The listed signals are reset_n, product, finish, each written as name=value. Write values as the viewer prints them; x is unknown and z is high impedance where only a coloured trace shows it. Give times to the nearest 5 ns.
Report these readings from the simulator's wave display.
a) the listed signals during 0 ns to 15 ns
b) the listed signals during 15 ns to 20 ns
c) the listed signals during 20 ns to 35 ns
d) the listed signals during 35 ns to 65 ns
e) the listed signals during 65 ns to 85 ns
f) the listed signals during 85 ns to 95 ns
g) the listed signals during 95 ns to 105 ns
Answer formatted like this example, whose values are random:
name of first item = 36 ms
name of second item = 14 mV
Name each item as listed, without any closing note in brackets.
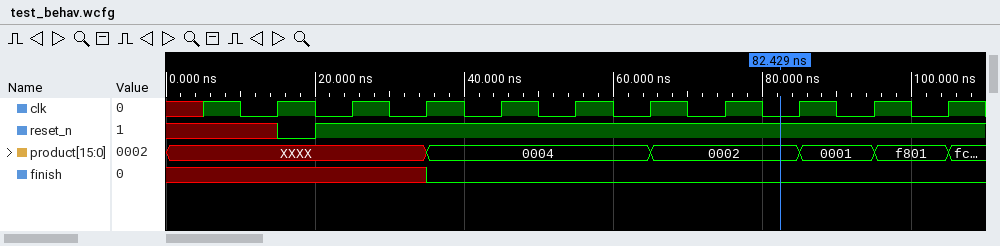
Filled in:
the listed signals during 0 ns to 15 ns = reset_n=x, product=XXXX, finish=x
the listed signals during 15 ns to 20 ns = reset_n=0, product=XXXX, finish=x
the listed signals during 20 ns to 35 ns = reset_n=1, product=XXXX, finish=x
the listed signals during 35 ns to 65 ns = reset_n=1, product=0004, finish=0
the listed signals during 65 ns to 85 ns = reset_n=1, product=0002, finish=0
the listed signals during 85 ns to 95 ns = reset_n=1, product=0001, finish=0
the listed signals during 95 ns to 105 ns = reset_n=1, product=f801, finish=0
